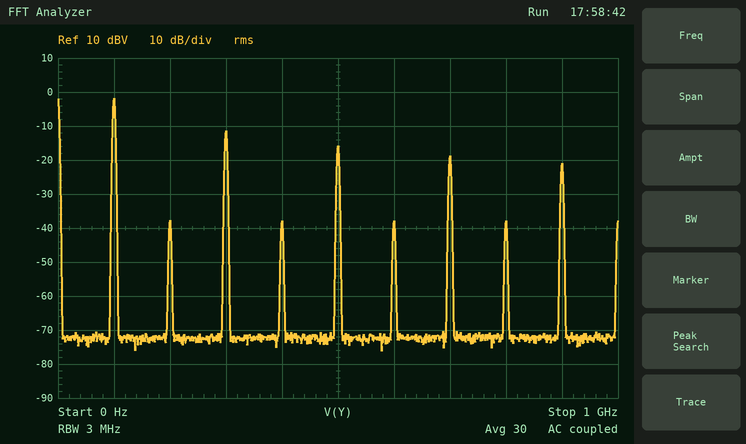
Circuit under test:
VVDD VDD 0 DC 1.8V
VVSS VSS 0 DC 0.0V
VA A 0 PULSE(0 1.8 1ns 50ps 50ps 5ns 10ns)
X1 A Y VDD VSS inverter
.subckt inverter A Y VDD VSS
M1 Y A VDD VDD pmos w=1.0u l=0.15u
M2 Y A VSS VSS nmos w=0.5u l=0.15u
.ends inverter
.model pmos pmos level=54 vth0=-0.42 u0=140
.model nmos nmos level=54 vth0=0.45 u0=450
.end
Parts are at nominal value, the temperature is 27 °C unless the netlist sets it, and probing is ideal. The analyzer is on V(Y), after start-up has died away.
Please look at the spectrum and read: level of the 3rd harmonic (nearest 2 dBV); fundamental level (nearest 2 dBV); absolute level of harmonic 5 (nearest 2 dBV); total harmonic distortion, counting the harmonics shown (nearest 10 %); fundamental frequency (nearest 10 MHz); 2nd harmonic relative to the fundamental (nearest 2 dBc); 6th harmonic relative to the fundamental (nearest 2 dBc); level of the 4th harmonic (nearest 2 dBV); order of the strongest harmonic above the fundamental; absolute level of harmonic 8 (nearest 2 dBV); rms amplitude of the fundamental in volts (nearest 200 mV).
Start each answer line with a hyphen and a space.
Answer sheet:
- -12 dBV
- -2 dBV
- -16 dBV
- 40 %
- 100 MHz
- -36 dBc
- -36 dBc
- -38 dBV
- 3
- -38 dBV
- 800 mV
